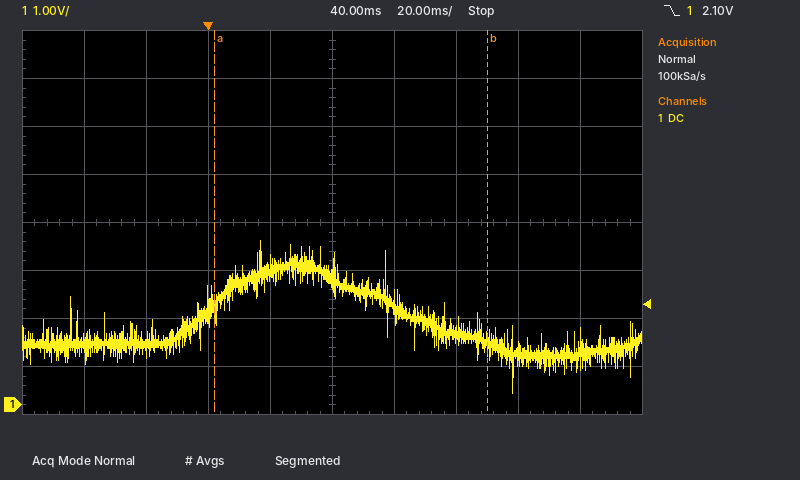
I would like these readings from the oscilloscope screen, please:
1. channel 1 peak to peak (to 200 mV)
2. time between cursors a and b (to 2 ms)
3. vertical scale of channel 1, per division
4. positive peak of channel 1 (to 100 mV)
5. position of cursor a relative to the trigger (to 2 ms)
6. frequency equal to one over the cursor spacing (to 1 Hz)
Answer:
3.2 V
88 ms
1 V
3.4 V
+2 ms
11 Hz
